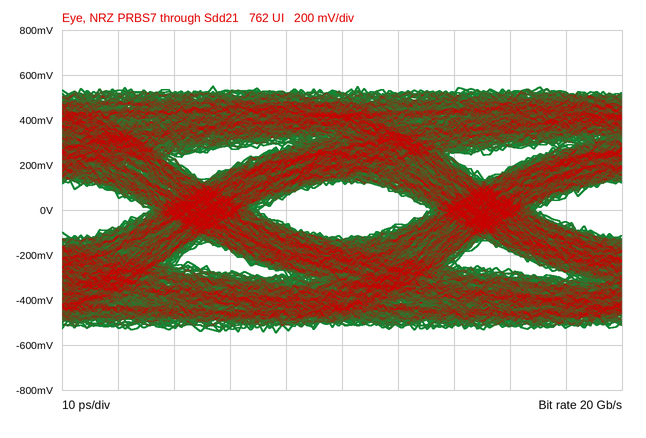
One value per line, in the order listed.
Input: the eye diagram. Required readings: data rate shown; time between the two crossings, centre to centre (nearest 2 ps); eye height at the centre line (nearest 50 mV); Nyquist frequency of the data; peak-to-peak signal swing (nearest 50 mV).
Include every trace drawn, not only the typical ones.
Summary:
20 Gb/s
50 ps
250 mV
10 GHz
1.10 V
